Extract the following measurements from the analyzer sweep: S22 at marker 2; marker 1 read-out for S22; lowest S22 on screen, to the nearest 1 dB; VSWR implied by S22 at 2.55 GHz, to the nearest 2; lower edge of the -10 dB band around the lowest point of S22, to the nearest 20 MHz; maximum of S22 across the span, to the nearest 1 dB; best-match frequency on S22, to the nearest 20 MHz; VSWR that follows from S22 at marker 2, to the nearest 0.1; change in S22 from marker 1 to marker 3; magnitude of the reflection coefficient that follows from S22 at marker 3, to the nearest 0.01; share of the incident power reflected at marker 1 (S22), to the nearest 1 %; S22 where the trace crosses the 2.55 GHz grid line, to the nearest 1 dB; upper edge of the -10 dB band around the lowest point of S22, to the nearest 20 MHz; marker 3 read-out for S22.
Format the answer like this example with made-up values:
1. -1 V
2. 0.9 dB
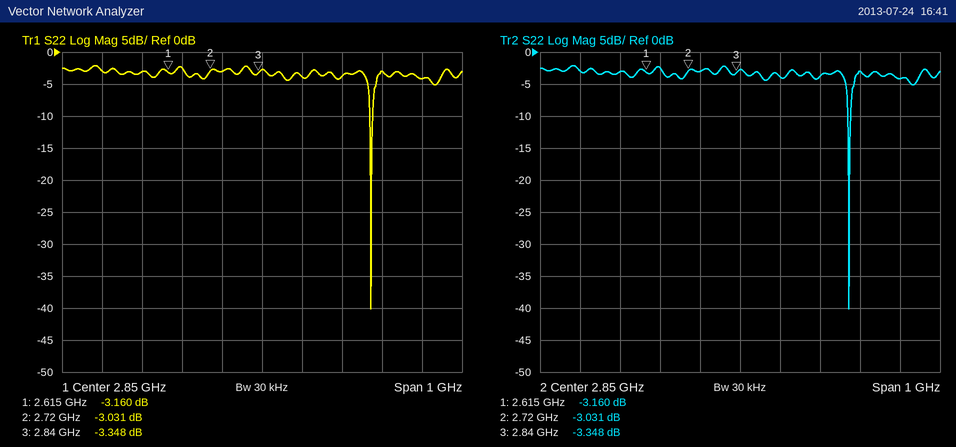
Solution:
1. -3.031 dB
2. -3.160 dB
3. -40 dB
4. 6
5. 3.12 GHz
6. -2 dB
7. 3.12 GHz
8. 5.8
9. -0.188 dB
10. 0.68
11. 48 %
12. -3 dB
13. 3.12 GHz
14. -3.348 dB
